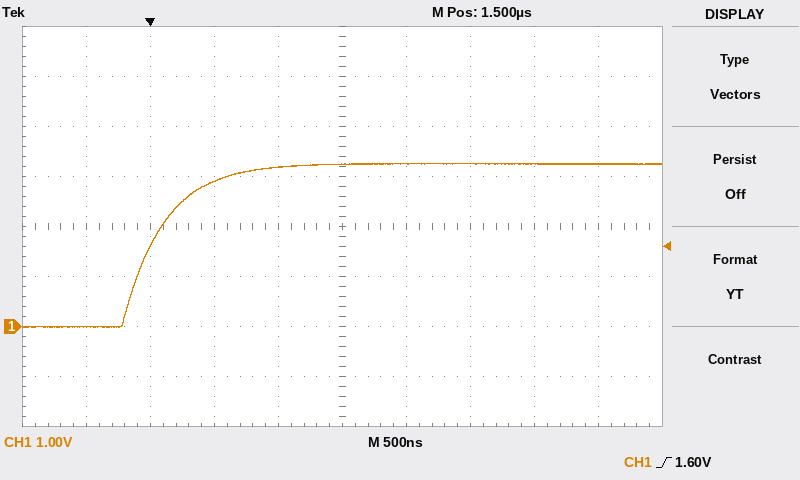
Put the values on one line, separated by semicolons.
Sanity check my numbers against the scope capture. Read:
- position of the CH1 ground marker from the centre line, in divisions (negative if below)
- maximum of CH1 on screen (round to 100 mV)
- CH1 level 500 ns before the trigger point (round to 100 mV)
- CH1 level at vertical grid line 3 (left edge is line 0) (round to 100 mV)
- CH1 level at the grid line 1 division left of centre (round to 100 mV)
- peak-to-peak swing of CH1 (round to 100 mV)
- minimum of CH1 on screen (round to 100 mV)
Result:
-2.0 div; 3.3 V; 0.0 V; 2.9 V; 3.2 V; 3.3 V; 0.0 V
